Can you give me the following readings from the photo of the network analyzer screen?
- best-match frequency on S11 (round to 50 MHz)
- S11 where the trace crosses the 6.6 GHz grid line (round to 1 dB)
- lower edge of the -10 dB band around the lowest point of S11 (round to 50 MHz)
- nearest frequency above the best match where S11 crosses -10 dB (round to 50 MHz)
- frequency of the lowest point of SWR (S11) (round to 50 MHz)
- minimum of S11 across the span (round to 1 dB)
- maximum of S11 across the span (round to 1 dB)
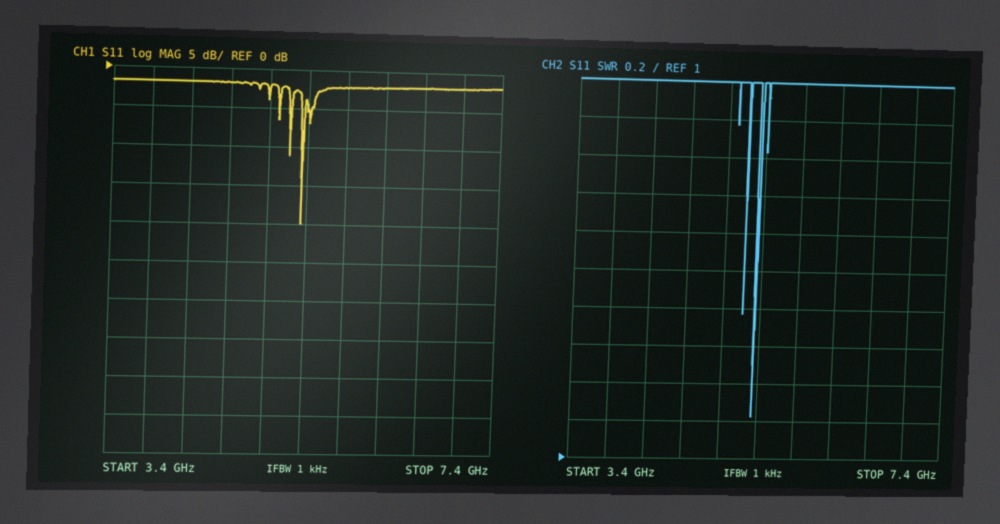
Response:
5.35 GHz
-2 dB
5.35 GHz
5.35 GHz
5.35 GHz
-20 dB
-2 dB
